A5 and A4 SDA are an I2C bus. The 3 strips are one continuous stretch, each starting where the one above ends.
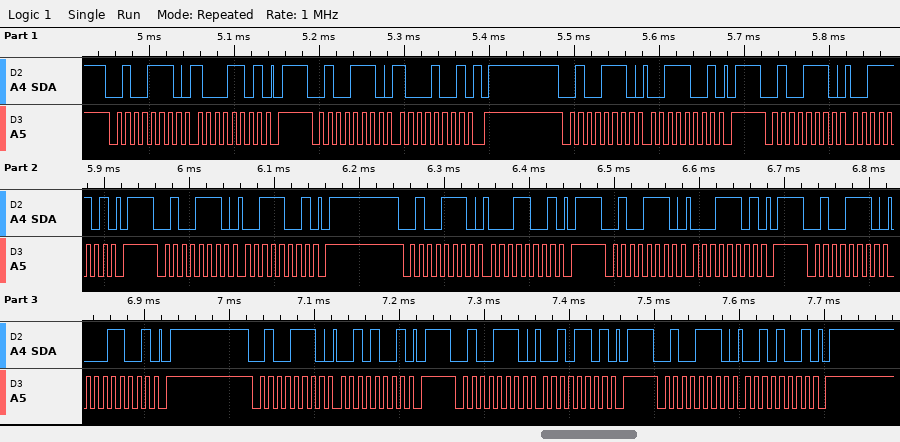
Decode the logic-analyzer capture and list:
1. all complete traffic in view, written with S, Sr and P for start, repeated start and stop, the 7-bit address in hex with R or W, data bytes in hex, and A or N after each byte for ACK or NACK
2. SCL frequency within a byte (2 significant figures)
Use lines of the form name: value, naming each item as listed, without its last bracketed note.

all complete traffic in view, written with S, Sr and P for start, repeated start and stop, the 7-bit address in hex with R or W, data bytes in hex, and A or N after each byte for ACK or NACK: S 27W A 8D A P S 27W A 89 A P S 27W A 39 A P S 27W A 3D A P S 27W A 39 A P S 27W A 19 A P S 27W A 1D A P S 27W A 19 A P S 27W A 29 A P S 27W A 2D A P S 27W A 29 A P
SCL frequency within a byte: 100 kHz
